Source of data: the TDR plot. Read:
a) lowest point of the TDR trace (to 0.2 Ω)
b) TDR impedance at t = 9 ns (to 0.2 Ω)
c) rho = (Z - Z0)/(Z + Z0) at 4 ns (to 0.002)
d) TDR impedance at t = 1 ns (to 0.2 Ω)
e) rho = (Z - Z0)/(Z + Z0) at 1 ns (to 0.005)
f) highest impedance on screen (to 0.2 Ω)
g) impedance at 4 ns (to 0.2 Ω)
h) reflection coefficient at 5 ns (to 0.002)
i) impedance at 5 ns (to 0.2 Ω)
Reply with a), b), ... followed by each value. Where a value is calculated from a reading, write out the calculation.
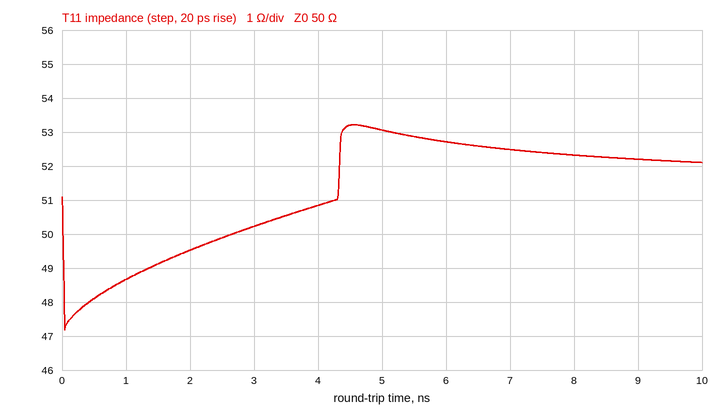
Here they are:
a) 47.2 Ω
b) 52.2 Ω
c) (50.8 − 50)/(50.8 + 50) ≈ +0.008
d) 48.6 Ω
e) (48.6 − 50)/(48.6 + 50) ≈ -0.0142, so -0.015 to the nearest 0.005
f) 53.2 Ω
g) 50.8 Ω
h) (53 − 50)/(53 + 50) ≈ +0.0291, so +0.030 to the nearest 0.002
i) 53.0 Ω
